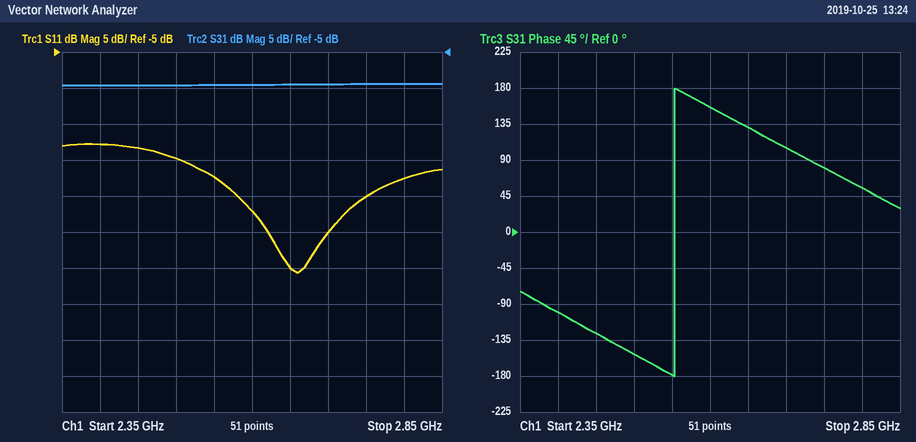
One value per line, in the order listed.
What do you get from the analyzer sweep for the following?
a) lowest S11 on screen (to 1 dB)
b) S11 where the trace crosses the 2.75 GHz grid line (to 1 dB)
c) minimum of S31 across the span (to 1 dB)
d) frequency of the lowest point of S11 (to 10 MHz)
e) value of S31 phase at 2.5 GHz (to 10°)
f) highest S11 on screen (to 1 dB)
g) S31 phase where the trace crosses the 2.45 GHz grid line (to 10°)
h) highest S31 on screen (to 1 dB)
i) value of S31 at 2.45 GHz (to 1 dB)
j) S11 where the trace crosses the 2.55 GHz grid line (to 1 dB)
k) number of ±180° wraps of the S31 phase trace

-36 dB
-25 dB
-10 dB
2.66 GHz
-150°
-18 dB
-130°
-9 dB
-10 dB
-22 dB
1
